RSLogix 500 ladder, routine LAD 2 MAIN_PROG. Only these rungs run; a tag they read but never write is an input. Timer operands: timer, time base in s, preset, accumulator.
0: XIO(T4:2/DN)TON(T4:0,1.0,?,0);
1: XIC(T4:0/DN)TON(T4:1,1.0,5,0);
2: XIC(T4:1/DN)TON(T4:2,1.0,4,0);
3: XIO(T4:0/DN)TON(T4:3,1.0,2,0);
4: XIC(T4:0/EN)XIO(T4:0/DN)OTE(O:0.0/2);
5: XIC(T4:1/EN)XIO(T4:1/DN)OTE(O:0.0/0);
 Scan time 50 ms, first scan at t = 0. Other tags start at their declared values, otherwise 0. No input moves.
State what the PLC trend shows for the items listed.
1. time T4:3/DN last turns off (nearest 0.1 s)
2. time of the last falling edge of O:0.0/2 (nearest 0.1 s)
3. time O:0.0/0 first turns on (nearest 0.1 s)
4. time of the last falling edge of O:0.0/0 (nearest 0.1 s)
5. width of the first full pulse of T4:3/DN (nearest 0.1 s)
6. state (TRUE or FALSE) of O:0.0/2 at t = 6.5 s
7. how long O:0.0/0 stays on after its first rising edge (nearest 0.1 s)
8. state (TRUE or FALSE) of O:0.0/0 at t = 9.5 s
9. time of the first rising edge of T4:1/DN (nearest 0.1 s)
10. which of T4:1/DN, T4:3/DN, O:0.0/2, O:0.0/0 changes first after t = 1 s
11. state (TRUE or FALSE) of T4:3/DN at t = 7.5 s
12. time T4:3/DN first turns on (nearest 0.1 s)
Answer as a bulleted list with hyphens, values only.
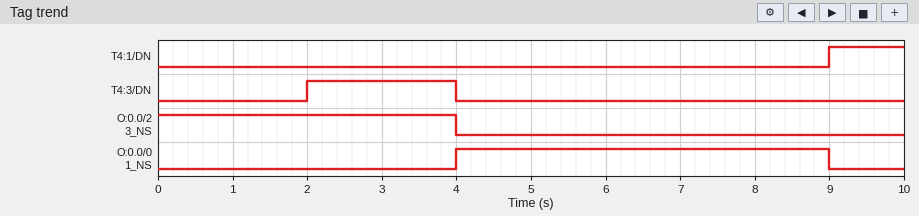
- 4.0 s
- 4.0 s
- 4.0 s
- 9.0 s
- 2.0 s
- FALSE
- 5.0 s
- FALSE
- 9.0 s
- T4:3/DN
- FALSE
- 2.0 s
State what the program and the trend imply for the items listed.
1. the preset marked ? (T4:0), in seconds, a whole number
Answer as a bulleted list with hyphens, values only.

- 4 s
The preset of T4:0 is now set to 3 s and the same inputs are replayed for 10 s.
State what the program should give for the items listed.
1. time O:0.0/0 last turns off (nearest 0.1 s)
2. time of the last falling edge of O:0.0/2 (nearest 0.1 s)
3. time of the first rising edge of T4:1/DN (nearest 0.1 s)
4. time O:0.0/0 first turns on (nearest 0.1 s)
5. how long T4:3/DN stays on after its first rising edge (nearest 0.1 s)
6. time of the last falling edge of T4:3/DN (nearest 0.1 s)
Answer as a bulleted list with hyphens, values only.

- 8.0 s
- 3.0 s
- 8.0 s
- 3.0 s
- 1.0 s
- 3.0 s
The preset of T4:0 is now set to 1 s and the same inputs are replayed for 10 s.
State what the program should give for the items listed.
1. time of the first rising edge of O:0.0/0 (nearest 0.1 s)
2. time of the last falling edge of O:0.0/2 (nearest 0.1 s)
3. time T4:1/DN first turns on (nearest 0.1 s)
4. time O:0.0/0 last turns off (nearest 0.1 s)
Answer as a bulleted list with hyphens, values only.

- 1.0 s
- 1.0 s
- 6.0 s
- 6.0 s
